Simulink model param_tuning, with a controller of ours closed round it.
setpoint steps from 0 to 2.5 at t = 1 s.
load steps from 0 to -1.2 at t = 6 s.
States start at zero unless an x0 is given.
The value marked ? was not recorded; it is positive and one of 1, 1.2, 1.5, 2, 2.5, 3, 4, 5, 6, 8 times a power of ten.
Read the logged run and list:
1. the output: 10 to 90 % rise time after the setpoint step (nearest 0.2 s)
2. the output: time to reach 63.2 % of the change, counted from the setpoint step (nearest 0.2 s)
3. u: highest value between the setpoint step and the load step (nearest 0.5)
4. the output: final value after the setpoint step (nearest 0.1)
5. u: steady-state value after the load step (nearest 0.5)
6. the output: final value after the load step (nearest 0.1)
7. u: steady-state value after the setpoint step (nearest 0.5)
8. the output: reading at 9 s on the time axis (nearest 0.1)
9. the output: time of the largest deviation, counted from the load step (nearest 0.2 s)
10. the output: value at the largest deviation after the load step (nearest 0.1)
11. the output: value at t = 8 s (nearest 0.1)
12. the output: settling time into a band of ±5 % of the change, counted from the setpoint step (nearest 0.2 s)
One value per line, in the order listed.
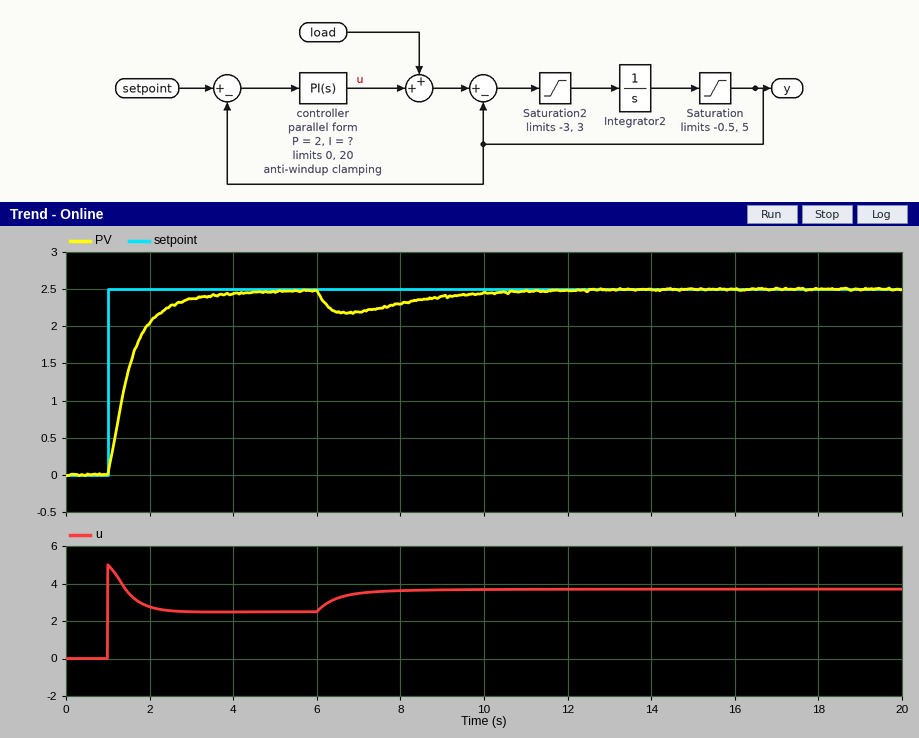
1.4 s
0.6 s
5.0
2.5
3.5
2.5
2.5
2.4
0.8 s
2.2
2.3
2.0 s
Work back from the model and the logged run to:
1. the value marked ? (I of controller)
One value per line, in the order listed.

1.5
